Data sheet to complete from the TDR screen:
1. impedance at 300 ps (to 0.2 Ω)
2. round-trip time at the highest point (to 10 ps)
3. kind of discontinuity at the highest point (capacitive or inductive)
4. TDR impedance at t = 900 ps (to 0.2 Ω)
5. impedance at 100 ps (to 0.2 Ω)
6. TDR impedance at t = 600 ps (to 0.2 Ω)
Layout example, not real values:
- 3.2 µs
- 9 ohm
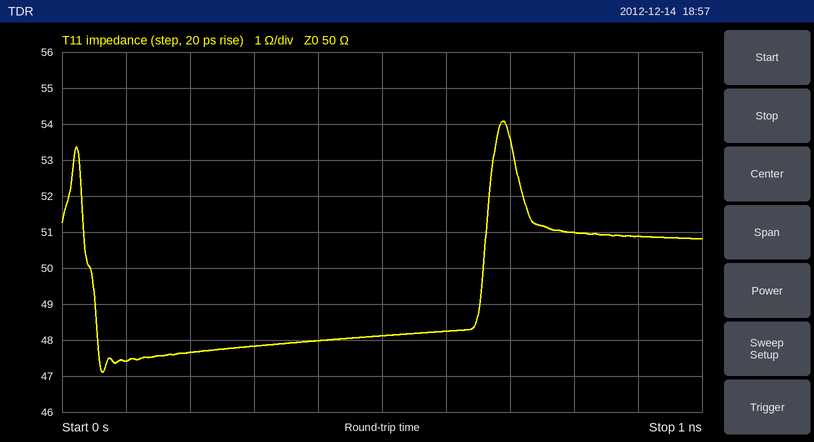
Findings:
- 47.8 Ω
- 690 ps
- inductive
- 50.8 Ω
- 47.4 Ω
- 48.2 Ω
